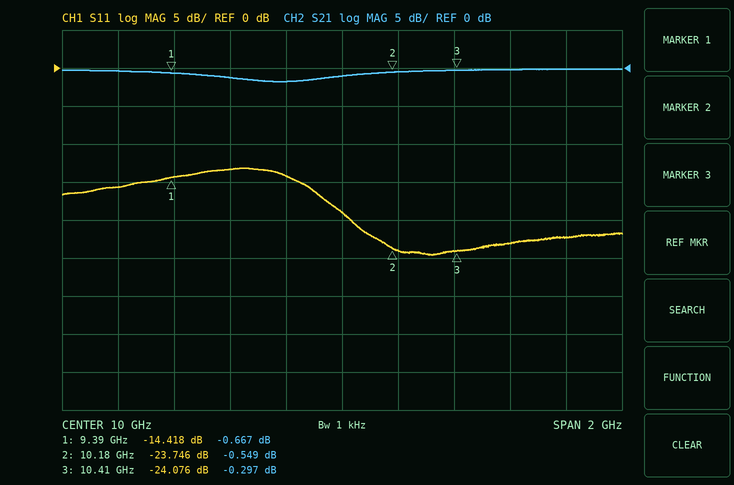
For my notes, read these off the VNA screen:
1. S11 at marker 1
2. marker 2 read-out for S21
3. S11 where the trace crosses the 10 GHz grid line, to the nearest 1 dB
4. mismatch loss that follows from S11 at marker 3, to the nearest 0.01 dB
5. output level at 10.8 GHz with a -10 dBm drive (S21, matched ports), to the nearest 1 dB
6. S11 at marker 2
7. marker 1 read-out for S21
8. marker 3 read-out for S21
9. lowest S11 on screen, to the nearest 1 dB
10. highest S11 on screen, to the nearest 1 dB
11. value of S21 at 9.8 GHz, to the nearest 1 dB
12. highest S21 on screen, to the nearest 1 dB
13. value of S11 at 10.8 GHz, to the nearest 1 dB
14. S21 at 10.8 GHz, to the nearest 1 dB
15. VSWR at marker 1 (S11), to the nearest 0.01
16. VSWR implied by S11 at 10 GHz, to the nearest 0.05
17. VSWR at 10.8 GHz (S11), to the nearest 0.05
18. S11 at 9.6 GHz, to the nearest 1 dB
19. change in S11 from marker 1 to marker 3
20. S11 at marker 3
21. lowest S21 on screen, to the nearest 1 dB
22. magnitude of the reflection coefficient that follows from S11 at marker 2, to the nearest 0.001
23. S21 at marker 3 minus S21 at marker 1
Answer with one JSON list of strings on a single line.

["-14.418 dB", "-0.549 dB", "-19 dB", "0.02 dB", "-10 dBm", "-23.746 dB", "-0.667 dB", "-0.297 dB", "-25 dB", "-13 dB", "-2 dB", "0 dB", "-22 dB", "0 dB", "1.47", "1.25", "1.15", "-13 dB", "-9.658 dB", "-24.076 dB", "-2 dB", "0.065", "0.370 dB"]
